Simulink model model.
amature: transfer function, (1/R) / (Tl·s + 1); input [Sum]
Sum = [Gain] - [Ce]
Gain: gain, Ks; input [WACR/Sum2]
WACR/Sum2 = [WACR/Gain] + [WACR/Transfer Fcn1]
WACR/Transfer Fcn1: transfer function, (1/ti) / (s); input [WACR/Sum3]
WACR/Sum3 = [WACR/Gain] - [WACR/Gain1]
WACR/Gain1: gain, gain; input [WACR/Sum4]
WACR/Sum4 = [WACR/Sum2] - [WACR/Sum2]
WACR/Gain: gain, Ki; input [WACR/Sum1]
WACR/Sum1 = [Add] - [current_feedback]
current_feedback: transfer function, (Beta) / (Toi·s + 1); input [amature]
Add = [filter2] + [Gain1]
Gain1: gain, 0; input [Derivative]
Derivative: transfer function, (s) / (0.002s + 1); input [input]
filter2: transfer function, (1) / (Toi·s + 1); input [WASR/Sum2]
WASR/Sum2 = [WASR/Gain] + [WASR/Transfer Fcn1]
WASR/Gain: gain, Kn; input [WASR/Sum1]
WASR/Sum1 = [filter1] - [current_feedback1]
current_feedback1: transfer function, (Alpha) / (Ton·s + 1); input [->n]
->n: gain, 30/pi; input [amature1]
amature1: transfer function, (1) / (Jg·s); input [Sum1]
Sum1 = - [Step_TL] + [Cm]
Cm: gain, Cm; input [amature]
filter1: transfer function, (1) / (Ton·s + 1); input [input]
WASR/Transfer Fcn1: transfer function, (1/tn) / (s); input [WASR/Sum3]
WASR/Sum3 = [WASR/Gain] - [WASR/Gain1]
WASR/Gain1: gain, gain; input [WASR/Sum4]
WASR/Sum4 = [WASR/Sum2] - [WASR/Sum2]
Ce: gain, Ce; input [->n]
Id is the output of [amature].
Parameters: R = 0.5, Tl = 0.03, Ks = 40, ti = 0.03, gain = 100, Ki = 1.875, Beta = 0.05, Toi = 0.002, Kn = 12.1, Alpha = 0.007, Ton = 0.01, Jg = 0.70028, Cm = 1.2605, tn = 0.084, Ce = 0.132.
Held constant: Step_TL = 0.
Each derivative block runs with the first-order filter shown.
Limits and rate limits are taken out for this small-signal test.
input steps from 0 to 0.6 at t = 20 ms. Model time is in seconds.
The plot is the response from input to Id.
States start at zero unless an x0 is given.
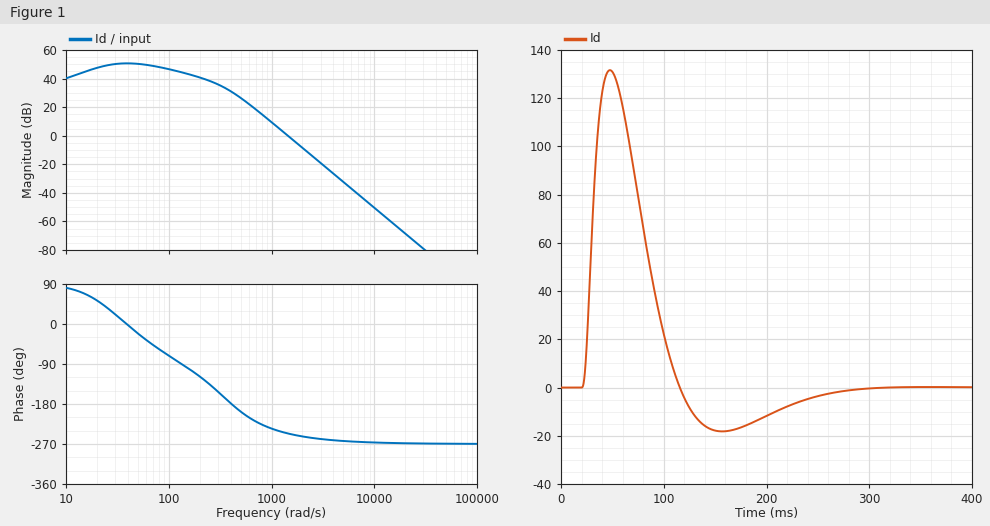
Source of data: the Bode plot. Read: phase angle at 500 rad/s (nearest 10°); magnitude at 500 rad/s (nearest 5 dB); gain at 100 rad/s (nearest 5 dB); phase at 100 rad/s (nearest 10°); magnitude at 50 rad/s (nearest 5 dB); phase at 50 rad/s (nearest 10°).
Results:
-200°
25 dB
45 dB
-70°
50 dB
-20°
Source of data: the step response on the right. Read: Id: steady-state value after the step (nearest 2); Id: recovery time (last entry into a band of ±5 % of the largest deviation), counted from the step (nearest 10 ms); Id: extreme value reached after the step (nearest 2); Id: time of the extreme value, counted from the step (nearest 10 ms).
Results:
0
210 ms
132
30 ms
